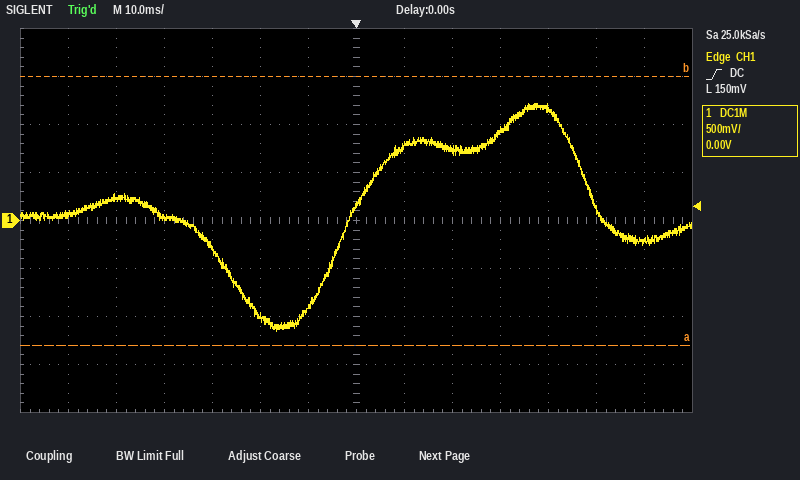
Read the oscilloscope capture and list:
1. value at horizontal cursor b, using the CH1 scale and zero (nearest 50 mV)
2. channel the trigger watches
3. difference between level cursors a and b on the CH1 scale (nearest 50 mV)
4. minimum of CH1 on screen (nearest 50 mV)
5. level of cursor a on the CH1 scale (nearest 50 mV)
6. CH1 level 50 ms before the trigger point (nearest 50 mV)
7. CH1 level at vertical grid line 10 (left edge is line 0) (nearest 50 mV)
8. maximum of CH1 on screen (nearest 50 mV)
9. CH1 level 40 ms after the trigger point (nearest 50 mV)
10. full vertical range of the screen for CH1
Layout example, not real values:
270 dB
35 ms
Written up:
1.50 V
CH1
2.80 V
-1.15 V
-1.30 V
250 mV
950 mV
1.20 V
1.15 V
4 V
